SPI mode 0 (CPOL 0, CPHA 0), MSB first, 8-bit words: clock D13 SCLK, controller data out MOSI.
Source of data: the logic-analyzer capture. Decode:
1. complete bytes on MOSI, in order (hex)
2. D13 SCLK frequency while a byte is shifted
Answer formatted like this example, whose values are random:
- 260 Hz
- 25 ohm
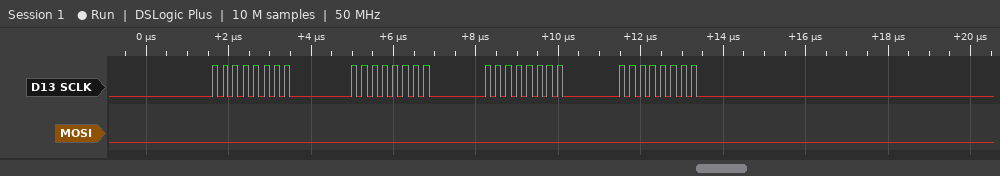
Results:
- 00 00 00 00
- 4 MHz
